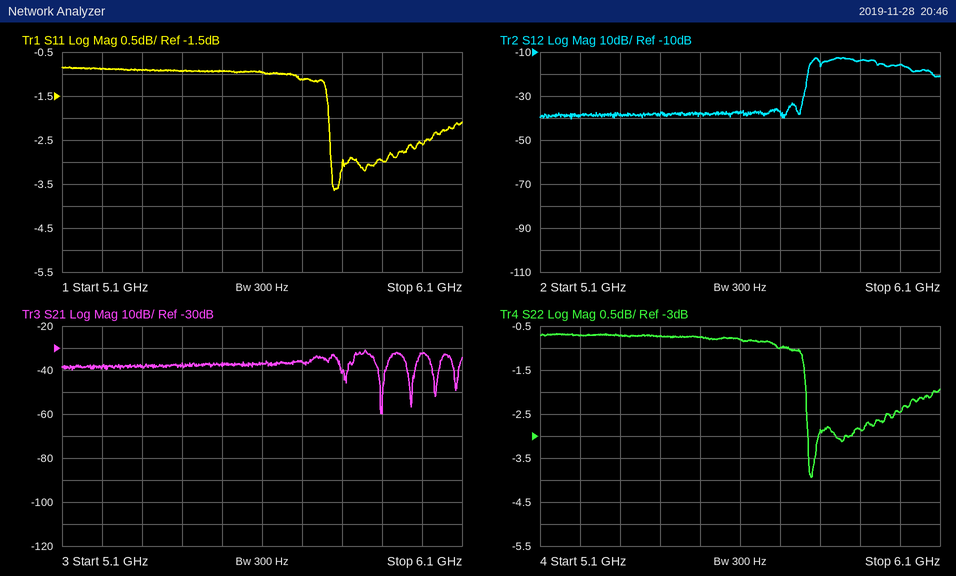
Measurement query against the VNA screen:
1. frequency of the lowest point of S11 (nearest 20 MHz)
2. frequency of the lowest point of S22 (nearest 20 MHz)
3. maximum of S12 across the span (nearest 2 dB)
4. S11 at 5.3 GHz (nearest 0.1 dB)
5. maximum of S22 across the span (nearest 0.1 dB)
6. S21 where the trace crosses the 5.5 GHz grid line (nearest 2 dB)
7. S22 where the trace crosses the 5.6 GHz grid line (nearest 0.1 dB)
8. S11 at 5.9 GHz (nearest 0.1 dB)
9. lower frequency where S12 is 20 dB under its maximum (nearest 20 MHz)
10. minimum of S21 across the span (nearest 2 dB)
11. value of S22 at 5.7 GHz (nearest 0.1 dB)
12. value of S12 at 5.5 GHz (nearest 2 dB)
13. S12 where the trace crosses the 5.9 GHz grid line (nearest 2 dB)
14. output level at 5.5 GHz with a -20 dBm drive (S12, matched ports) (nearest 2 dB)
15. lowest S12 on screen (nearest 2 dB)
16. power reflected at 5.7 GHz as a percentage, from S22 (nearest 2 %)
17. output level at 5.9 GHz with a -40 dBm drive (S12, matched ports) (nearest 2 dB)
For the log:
5.78 GHz
5.78 GHz
-12 dB
-0.9 dB
-0.7 dB
-38 dB
-0.8 dB
-3.0 dB
5.76 GHz
-60 dB
-1.0 dB
-38 dB
-14 dB
-58 dBm
-40 dB
80 %
-54 dBm
